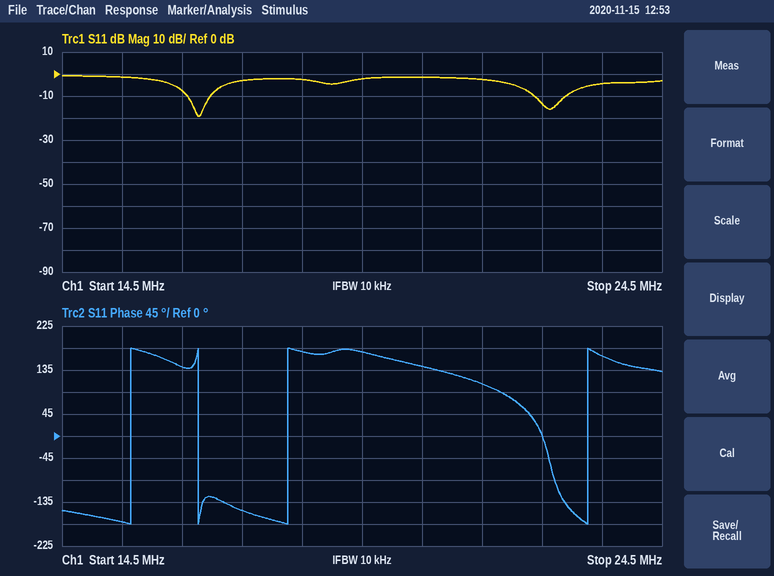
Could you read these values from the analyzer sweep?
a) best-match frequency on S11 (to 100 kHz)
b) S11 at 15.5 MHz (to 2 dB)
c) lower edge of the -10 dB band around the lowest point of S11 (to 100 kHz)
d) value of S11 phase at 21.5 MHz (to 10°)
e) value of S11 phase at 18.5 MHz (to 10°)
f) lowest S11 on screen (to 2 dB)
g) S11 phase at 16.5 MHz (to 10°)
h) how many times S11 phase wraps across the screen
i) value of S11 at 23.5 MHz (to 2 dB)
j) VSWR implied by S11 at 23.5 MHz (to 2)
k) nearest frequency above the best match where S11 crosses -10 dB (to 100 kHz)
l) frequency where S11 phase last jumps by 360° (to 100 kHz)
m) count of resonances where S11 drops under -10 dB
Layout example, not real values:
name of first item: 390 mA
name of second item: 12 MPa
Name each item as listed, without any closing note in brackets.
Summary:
best-match frequency on S11: 16.8 MHz
S11 at 15.5 MHz: -2 dB
lower edge of the -10 dB band around the lowest point of S11: 16.6 MHz
value of S11 phase at 21.5 MHz: 110°
value of S11 phase at 18.5 MHz: 170°
lowest S11 on screen: -20 dB
S11 phase at 16.5 MHz: 140°
how many times S11 phase wraps across the screen: 4
value of S11 at 23.5 MHz: -4 dB
VSWR implied by S11 at 23.5 MHz: 4
nearest frequency above the best match where S11 crosses -10 dB: 17.0 MHz
frequency where S11 phase last jumps by 360°: 23.3 MHz
count of resonances where S11 drops under -10 dB: 2
